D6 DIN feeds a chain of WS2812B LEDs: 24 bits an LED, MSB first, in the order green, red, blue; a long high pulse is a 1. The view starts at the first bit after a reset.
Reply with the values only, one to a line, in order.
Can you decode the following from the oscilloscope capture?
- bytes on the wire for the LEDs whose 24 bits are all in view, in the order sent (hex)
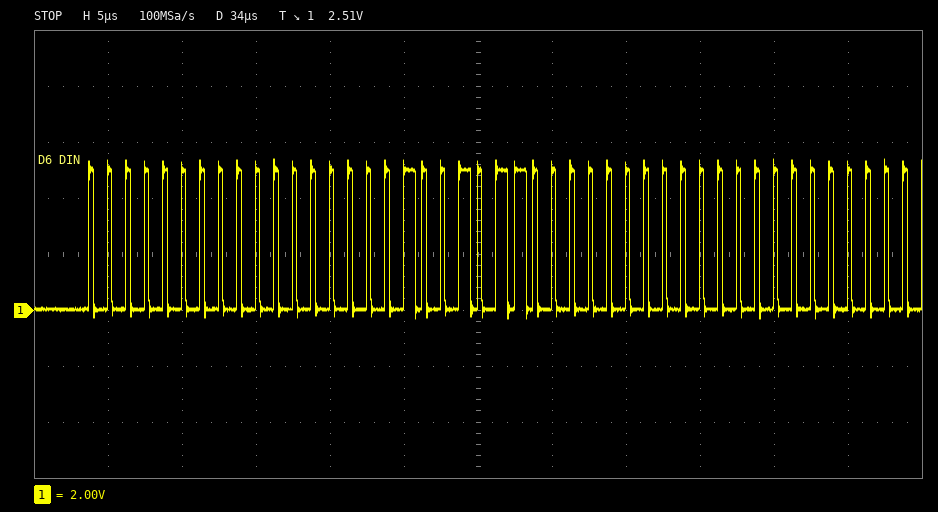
00 00 4B
